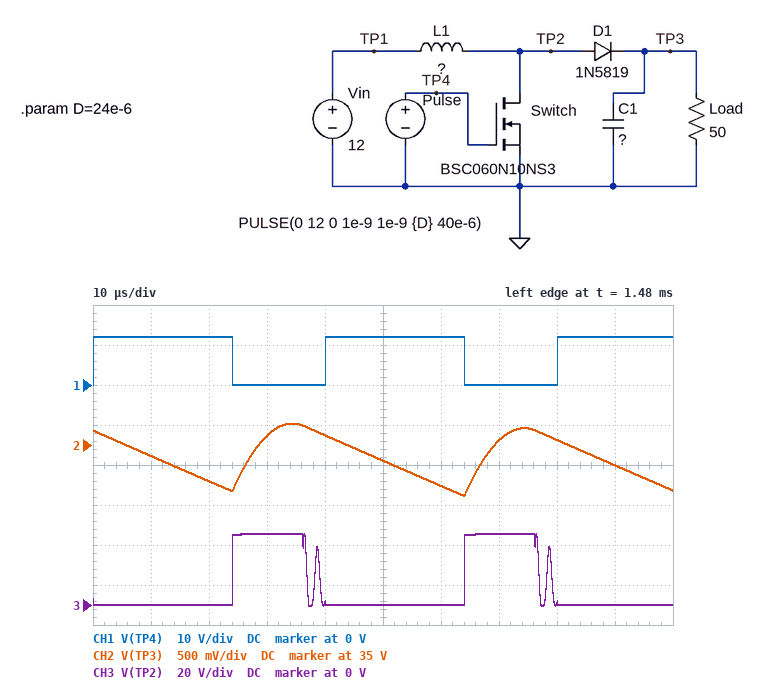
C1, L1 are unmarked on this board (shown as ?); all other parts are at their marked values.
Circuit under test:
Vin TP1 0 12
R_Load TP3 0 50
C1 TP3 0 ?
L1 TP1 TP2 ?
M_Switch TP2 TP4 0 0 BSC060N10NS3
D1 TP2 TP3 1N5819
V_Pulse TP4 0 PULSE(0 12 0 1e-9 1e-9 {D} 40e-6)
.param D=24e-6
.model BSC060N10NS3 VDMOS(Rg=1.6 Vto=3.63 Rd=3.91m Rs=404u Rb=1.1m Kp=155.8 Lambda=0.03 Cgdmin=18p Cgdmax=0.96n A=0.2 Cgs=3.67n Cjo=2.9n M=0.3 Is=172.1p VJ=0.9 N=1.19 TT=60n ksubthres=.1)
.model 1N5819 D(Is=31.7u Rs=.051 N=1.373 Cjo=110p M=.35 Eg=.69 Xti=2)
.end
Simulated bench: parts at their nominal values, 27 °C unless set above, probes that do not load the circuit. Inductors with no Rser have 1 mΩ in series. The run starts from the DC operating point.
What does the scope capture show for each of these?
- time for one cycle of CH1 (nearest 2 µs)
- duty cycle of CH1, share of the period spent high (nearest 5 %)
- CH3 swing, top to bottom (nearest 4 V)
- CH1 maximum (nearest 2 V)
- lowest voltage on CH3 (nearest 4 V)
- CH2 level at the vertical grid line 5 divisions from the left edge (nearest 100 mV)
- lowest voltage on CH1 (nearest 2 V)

40 µs
60 %
36 V
12 V
0 V
34.8 V
0 V
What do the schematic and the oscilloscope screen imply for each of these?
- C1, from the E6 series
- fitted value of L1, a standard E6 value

22 µF
68 µH
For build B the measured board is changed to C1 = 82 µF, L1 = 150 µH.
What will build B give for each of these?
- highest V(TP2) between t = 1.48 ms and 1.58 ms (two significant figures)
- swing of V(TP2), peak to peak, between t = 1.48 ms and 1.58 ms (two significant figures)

40 V
41 V
